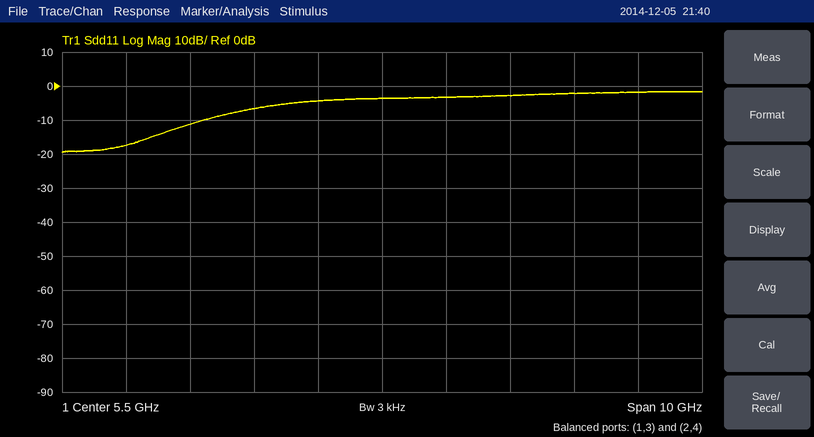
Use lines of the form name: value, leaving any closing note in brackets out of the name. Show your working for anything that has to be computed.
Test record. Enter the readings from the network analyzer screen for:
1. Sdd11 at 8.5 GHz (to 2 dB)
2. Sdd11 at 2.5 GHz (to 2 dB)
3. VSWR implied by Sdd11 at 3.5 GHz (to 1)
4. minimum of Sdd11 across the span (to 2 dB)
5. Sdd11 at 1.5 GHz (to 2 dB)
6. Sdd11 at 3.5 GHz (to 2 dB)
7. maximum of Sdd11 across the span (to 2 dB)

Sdd11 at 8.5 GHz: -2 dB
Sdd11 at 2.5 GHz: -12 dB
VSWR implied by Sdd11 at 3.5 GHz: |Γ| = 10^(-6/20) = 0.5012; VSWR = (1 + 0.5012)/(1 − 0.5012) ≈ 3
minimum of Sdd11 across the span: -20 dB
Sdd11 at 1.5 GHz: -18 dB
Sdd11 at 3.5 GHz: -6 dB
maximum of Sdd11 across the span: -2 dB
